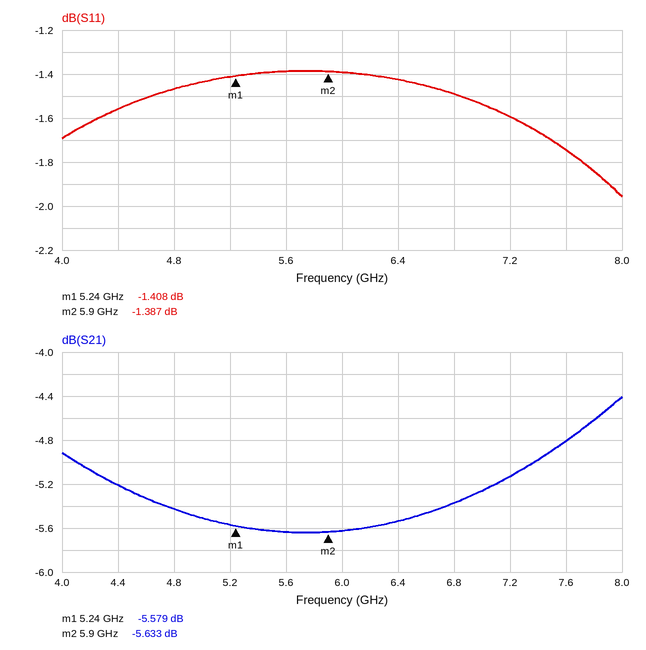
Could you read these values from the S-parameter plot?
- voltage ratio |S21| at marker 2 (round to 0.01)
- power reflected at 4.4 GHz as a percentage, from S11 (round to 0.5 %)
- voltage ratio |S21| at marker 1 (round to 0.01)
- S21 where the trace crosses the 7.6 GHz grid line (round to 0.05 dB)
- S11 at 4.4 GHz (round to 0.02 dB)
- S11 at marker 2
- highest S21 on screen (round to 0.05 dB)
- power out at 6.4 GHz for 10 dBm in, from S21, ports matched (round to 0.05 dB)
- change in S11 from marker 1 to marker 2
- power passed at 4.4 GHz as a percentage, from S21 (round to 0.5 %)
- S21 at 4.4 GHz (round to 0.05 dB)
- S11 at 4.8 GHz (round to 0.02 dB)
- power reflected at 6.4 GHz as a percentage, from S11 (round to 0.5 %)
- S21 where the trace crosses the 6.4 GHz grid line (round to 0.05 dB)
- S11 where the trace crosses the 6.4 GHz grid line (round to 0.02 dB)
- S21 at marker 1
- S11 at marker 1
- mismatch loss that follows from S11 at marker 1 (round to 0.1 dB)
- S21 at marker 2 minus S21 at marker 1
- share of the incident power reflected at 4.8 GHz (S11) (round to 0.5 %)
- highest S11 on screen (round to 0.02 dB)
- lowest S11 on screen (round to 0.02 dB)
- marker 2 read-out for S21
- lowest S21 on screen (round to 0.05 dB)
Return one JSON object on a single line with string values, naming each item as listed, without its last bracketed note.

{"voltage ratio |S21| at marker 2": "0.52", "power reflected at 4.4 GHz as a percentage, from S11": "70.0 %", "voltage ratio |S21| at marker 1": "0.53", "S21 where the trace crosses the 7.6 GHz grid line": "-4.80 dB", "S11 at 4.4 GHz": "-1.56 dB", "S11 at marker 2": "-1.387 dB", "highest S21 on screen": "-4.40 dB", "power out at 6.4 GHz for 10 dBm in, from S21, ports matched": "4.45 dBm", "change in S11 from marker 1 to marker 2": "0.021 dB", "power passed at 4.4 GHz as a percentage, from S21": "30.0 %", "S21 at 4.4 GHz": "-5.20 dB", "S11 at 4.8 GHz": "-1.46 dB", "power reflected at 6.4 GHz as a percentage, from S11": "72.0 %", "S21 where the trace crosses the 6.4 GHz grid line": "-5.55 dB", "S11 where the trace crosses the 6.4 GHz grid line": "-1.42 dB", "S21 at marker 1": "-5.579 dB", "S11 at marker 1": "-1.408 dB", "mismatch loss that follows from S11 at marker 1": "5.6 dB", "S21 at marker 2 minus S21 at marker 1": "-0.054 dB", "share of the incident power reflected at 4.8 GHz (S11)": "71.5 %", "highest S11 on screen": "-1.38 dB", "lowest S11 on screen": "-1.96 dB", "marker 2 read-out for S21": "-5.633 dB", "lowest S21 on screen": "-5.65 dB"}
